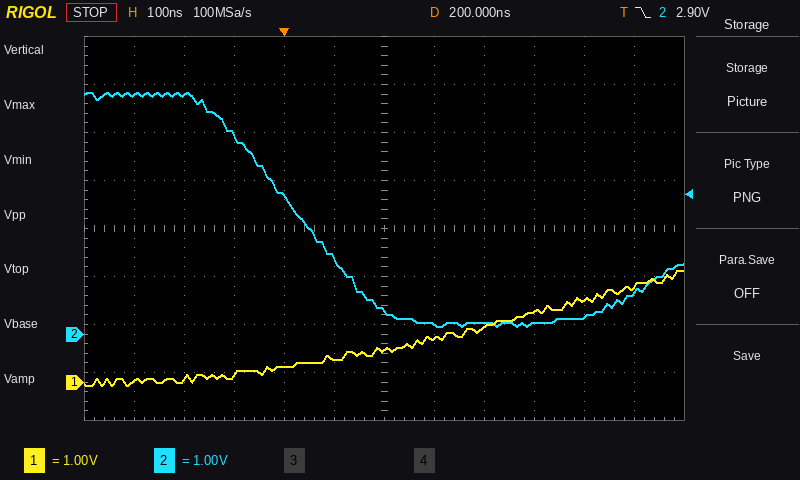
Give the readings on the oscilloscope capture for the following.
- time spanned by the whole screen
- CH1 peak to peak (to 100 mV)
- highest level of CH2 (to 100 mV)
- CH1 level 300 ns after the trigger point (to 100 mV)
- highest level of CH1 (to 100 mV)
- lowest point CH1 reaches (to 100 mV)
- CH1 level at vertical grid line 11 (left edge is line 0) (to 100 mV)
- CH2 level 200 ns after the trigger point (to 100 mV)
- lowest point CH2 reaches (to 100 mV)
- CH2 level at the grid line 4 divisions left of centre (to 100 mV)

1.2 µs
2.4 V
5.0 V
900 mV
2.3 V
-100 mV
2.0 V
500 mV
200 mV
5.0 V
